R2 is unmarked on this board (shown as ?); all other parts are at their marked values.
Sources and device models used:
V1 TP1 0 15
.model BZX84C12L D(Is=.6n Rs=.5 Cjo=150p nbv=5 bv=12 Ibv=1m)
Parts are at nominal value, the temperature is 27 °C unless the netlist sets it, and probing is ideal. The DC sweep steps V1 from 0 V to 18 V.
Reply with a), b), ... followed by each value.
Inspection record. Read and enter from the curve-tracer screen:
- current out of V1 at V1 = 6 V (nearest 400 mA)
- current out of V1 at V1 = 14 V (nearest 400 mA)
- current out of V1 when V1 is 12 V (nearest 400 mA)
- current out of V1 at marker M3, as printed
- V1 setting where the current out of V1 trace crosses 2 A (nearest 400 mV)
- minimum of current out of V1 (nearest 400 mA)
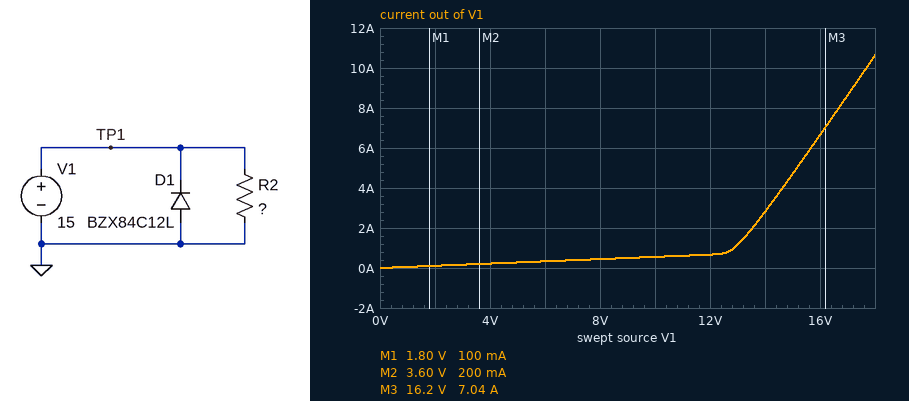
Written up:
a) 400 mA
b) 2.8 A
c) 800 mA
d) 7.04 A
e) 13.6 V
f) 0 A
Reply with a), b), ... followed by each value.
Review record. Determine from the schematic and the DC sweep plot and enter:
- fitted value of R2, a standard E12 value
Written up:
a) 18 Ω
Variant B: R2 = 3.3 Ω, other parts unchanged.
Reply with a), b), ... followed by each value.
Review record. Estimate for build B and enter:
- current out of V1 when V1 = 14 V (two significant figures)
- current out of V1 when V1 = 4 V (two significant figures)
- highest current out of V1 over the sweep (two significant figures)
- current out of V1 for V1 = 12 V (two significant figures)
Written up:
a) 6.3 A
b) 1.2 A
c) 15 A
d) 3.6 A
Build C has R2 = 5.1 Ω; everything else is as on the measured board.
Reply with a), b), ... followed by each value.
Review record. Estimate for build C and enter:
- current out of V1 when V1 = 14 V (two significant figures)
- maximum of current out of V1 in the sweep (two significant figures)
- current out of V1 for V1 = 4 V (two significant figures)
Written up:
a) 4.8 A
b) 13 A
c) 780 mA
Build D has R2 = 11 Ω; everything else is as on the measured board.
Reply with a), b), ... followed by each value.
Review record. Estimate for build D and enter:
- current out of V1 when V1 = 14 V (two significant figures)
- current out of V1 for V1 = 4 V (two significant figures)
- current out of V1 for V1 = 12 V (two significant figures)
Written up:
a) 3.3 A
b) 360 mA
c) 1.1 A
